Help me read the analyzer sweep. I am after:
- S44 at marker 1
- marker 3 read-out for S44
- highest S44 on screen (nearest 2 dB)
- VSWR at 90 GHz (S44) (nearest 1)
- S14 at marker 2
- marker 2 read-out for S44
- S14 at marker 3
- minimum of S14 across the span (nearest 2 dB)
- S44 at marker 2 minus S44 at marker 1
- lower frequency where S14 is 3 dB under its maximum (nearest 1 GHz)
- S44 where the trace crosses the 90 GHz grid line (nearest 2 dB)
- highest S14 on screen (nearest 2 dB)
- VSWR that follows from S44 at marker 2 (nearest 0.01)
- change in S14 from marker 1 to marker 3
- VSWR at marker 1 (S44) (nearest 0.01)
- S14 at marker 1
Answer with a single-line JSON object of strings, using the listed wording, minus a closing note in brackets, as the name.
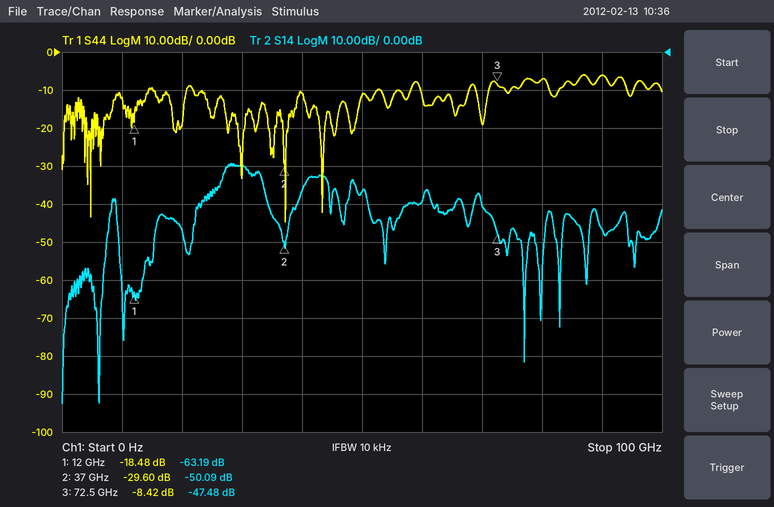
{"S44 at marker 1": "-18.48 dB", "marker 3 read-out for S44": "-8.42 dB", "highest S44 on screen": "-6 dB", "VSWR at 90 GHz (S44)": "3", "S14 at marker 2": "-50.09 dB", "marker 2 read-out for S44": "-29.60 dB", "S14 at marker 3": "-47.48 dB", "minimum of S14 across the span": "-92 dB", "S44 at marker 2 minus S44 at marker 1": "-11.12 dB", "lower frequency where S14 is 3 dB under its maximum": "27 GHz", "S44 where the trace crosses the 90 GHz grid line": "-6 dB", "highest S14 on screen": "-30 dB", "VSWR that follows from S44 at marker 2": "1.07", "change in S14 from marker 1 to marker 3": "15.71 dB", "VSWR at marker 1 (S44)": "1.27", "S14 at marker 1": "-63.19 dB"}
